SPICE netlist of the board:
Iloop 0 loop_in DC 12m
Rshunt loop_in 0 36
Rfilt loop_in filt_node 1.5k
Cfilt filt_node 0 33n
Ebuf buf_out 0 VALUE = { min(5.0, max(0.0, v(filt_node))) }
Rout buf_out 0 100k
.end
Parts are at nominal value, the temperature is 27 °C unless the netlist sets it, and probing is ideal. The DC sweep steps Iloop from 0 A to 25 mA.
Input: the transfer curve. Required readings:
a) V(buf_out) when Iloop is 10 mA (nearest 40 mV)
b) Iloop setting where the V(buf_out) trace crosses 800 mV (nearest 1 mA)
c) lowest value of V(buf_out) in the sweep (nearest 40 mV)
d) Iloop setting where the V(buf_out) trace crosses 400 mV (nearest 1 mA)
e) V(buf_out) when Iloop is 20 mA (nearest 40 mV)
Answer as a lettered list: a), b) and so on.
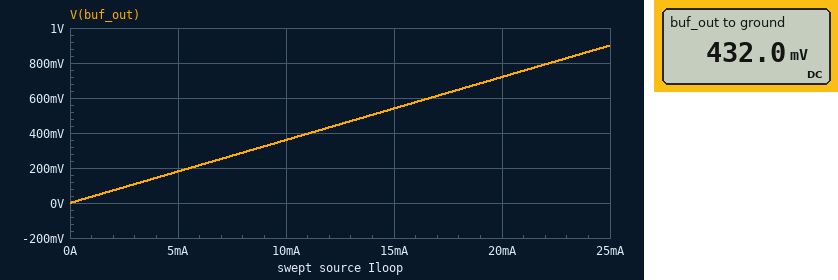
a) 360 mV
b) 22 mA
c) 0 V
d) 11 mA
e) 720 mV
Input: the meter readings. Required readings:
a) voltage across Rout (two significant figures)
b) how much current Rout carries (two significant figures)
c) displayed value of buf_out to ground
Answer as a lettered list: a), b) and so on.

a) 430 mV
b) 4.3 µA
c) 432.0 mV
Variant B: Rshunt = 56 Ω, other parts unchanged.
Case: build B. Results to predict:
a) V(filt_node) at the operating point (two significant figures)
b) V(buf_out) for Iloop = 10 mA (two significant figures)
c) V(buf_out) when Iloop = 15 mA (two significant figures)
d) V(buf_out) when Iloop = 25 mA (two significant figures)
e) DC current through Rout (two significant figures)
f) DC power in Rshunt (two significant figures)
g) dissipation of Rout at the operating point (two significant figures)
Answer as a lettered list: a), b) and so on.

a) 670 mV
b) 560 mV
c) 840 mV
d) 1.4 V
e) 6.7 µA
f) 8.1 mW
g) 4.5 µW
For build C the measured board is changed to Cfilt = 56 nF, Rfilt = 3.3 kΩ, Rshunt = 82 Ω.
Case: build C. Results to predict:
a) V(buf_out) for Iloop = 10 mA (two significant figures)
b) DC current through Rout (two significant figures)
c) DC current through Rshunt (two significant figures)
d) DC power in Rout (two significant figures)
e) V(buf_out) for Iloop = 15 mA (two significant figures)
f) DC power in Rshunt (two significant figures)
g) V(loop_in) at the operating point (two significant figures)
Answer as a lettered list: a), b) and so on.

a) 820 mV
b) 9.8 µA
c) 12 mA
d) 9.7 µW
e) 1.2 V
f) 12 mW
g) 980 mV
